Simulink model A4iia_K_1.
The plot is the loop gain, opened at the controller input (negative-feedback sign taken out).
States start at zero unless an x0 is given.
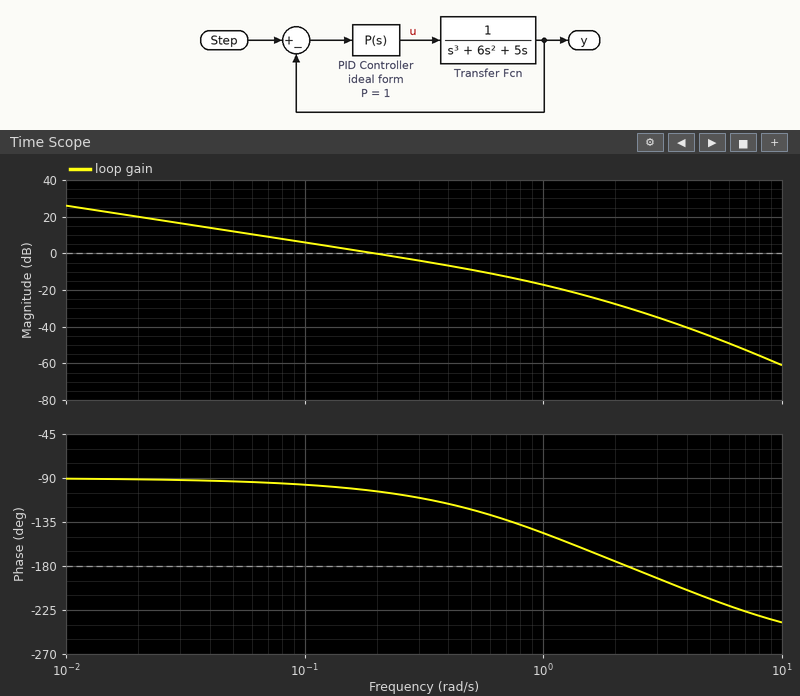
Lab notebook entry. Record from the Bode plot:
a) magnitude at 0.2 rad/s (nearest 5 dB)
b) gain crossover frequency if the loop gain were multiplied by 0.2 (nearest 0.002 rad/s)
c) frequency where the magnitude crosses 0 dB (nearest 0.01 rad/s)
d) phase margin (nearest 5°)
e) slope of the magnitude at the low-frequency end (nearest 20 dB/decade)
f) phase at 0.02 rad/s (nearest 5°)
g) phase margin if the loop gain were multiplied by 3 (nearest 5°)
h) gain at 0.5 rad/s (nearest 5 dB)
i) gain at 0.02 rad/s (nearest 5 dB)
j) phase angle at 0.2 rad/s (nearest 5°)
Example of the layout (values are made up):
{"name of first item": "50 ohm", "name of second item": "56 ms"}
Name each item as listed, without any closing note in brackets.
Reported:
{"magnitude at 0.2 rad/s": "0 dB", "gain crossover frequency if the loop gain were multiplied by 0.2": "0.040 rad/s", "frequency where the magnitude crosses 0 dB": "0.20 rad/s", "phase margin": "75°", "slope of the magnitude at the low-frequency end": "-20 dB/decade", "phase at 0.02 rad/s": "-90°", "phase margin if the loop gain were multiplied by 3": "55°", "gain at 0.5 rad/s": "-10 dB", "gain at 0.02 rad/s": "20 dB", "phase angle at 0.2 rad/s": "-105°"}
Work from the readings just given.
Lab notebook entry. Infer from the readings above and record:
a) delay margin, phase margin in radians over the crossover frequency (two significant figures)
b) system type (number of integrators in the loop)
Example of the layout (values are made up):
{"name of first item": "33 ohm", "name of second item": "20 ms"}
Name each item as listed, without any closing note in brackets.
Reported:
{"delay margin, phase margin in radians over the crossover frequency": "6.5 s", "system type": "1"}
